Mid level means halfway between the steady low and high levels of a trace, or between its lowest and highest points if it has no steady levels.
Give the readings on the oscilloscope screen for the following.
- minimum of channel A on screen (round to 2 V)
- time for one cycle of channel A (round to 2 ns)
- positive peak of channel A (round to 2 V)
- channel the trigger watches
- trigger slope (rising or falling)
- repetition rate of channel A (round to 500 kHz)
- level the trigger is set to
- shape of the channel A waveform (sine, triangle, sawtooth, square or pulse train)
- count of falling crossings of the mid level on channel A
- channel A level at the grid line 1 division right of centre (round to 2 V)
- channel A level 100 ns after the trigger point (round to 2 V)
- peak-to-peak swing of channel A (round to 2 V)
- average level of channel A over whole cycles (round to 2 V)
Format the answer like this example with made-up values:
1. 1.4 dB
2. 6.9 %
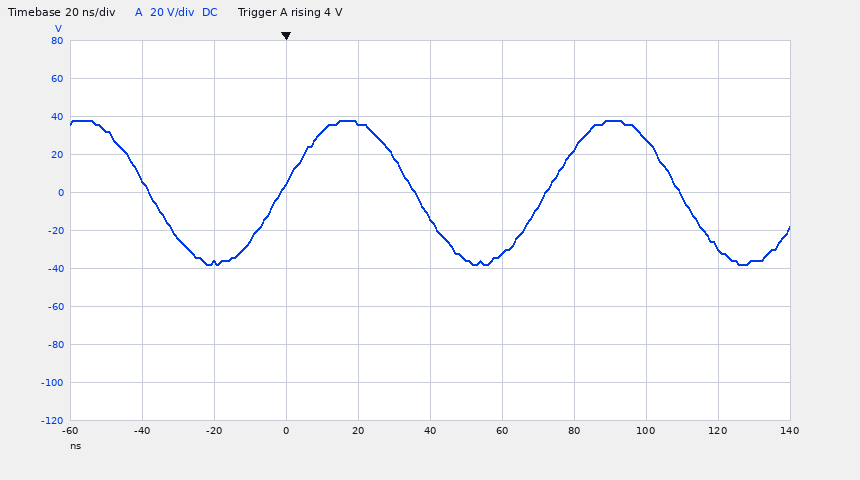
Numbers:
1. -38 V
2. 74 ns
3. 38 V
4. channel A
5. rising
6. 13.5 MHz
7. 4 V
8. sine
9. 3
10. -32 V
11. 28 V
12. 76 V
13. 0 V
